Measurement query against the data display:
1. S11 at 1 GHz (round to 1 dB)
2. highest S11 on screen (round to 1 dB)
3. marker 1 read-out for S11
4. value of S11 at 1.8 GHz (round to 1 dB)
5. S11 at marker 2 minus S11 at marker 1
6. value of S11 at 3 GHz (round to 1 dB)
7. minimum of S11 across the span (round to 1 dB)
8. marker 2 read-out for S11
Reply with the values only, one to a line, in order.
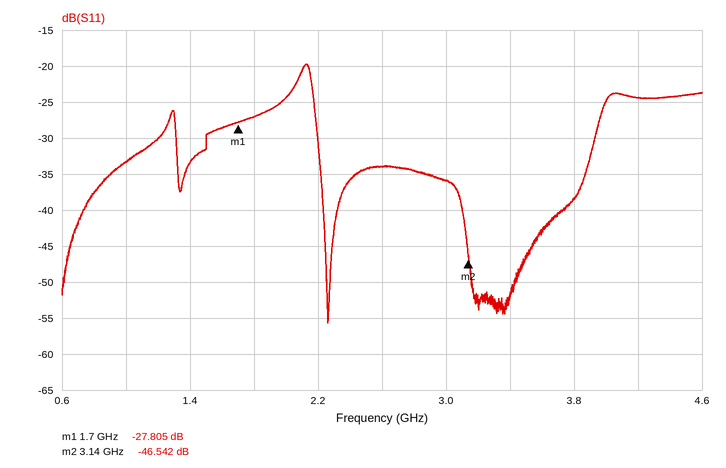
-33 dB
-20 dB
-27.805 dB
-27 dB
-18.737 dB
-36 dB
-56 dB
-46.542 dB
